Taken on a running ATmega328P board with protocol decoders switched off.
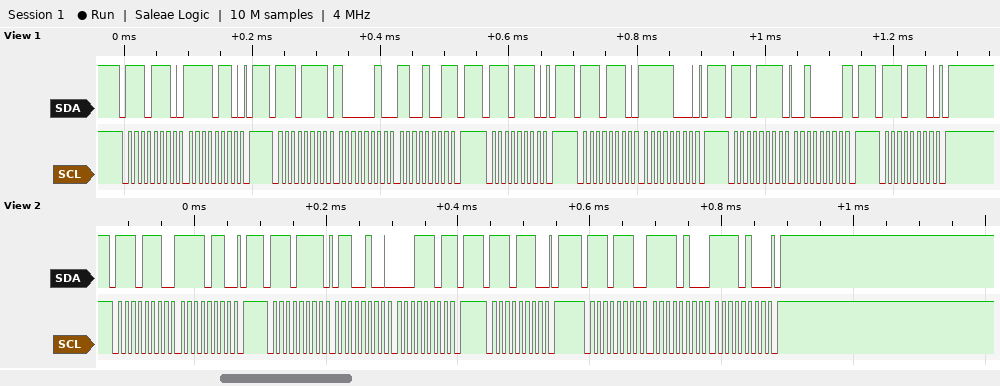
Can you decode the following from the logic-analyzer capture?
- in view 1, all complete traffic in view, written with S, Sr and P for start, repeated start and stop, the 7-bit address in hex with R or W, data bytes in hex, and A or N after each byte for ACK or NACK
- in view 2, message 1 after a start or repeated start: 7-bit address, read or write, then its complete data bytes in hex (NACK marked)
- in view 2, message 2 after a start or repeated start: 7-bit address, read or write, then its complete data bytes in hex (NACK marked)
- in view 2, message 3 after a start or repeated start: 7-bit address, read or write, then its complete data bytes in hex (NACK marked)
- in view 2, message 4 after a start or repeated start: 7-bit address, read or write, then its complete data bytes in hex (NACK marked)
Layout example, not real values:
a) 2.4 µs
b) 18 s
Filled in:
a) S 77W A F6 A P S 77R A 82 A C9 N P S 77W A P S 77W A F8 A P S 77R A 20 N P S 77W A P
b) 0x77 write: F6
c) 0x77 read: 64 1D NACK
d) 0x77 write
e) 0x77 write: F4 F4
